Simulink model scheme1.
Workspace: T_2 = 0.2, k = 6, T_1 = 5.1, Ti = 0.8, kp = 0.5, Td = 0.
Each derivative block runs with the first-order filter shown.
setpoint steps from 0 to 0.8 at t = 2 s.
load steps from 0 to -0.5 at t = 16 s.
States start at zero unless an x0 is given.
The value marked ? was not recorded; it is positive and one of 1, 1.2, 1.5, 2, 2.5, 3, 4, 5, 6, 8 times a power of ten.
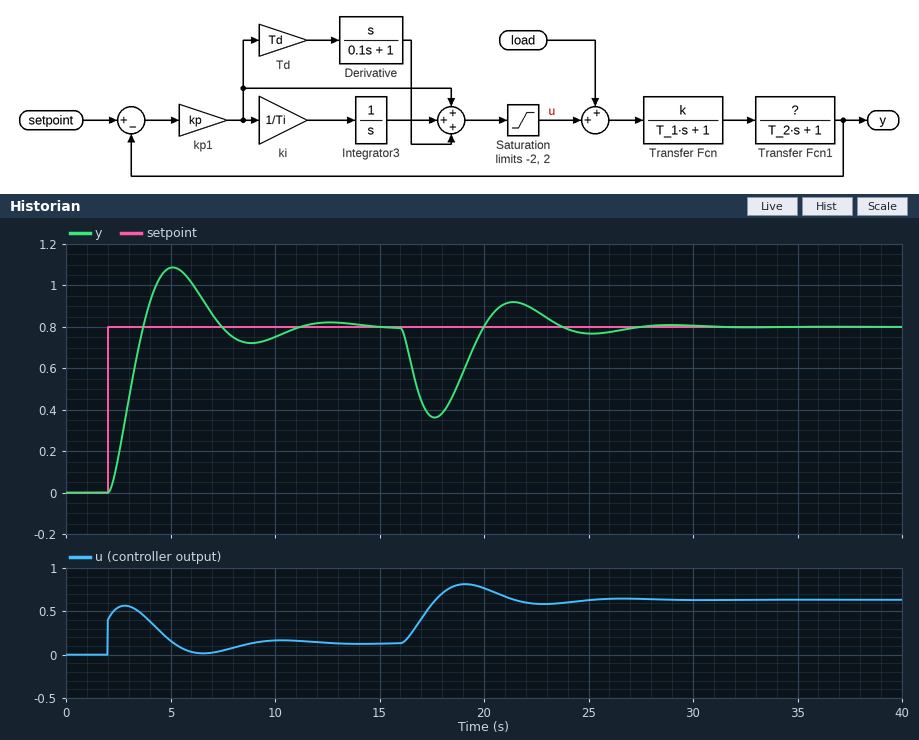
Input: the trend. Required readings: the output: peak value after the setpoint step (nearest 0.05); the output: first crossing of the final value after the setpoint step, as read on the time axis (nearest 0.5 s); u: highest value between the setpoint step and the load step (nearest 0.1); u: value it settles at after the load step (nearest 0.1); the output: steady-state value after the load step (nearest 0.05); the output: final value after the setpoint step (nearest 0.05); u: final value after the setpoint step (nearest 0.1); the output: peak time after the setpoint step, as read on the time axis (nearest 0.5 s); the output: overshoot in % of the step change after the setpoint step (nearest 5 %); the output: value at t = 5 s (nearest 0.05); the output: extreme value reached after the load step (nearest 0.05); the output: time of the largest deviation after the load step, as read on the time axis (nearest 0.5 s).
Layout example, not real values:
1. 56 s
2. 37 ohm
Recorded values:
1. 1.10
2. 3.5 s
3. 0.6
4. 0.6
5. 0.80
6. 0.80
7. 0.1
8. 5.0 s
9. 35 %
10. 1.10
11. 0.35
12. 17.5 s
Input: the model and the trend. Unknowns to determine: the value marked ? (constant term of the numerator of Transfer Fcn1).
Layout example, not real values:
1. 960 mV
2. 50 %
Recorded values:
1. 1
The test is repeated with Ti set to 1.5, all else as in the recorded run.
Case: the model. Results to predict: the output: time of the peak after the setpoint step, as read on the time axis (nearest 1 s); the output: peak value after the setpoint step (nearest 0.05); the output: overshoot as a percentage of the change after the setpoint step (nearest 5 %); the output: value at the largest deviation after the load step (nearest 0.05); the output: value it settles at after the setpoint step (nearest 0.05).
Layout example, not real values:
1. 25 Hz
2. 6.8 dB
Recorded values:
1. 6 s
2. 0.95
3. 20 %
4. 0.30
5. 0.80
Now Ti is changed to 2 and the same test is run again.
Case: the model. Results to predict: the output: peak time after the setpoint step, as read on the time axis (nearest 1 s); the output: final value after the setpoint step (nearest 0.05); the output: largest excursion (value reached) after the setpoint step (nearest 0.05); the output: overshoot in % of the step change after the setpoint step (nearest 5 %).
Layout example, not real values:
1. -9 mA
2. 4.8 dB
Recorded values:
1. 7 s
2. 0.80
3. 0.90
4. 15 %
